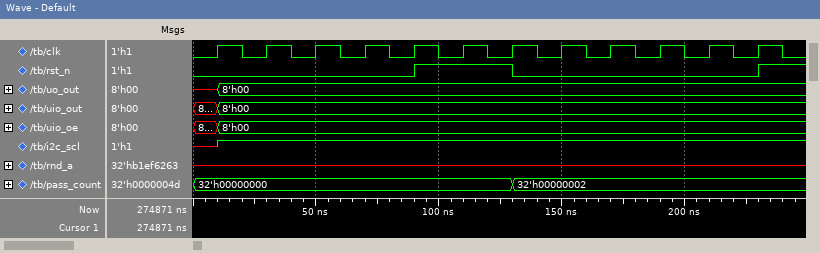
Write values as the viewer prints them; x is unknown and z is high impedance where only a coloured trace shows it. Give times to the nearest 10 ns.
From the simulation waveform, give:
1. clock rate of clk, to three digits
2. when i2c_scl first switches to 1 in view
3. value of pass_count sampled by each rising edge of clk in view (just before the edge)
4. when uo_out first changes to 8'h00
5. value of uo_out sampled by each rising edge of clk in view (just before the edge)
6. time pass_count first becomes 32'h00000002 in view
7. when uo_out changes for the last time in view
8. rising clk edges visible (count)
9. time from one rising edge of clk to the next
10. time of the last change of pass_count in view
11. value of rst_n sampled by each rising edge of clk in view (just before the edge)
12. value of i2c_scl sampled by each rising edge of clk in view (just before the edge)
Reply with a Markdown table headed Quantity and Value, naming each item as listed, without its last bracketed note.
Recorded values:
| Quantity | Value |
|---|---|
| clock rate of clk, to three digits | 50.0 MHz |
| when i2c_scl first switches to 1 in view | 10 ns |
| value of pass_count sampled by each rising edge of clk in view | 32'h00000000, 32'h00000000, 32'h00000000, 32'h00000000, 32'h00000000, 32'h00000000, 32'h00000000, 32'h00000002, 32'h00000002, 32'h00000002, 32'h00000002, 32'h00000002 |
| when uo_out first changes to 8'h00 | 10 ns |
| value of uo_out sampled by each rising edge of clk in view | x, 8'h00, 8'h00, 8'h00, 8'h00, 8'h00, 8'h00, 8'h00, 8'h00, 8'h00, 8'h00, 8'h00 |
| time pass_count first becomes 32'h00000002 in view | 130 ns |
| when uo_out changes for the last time in view | 10 ns |
| rising clk edges visible | 12 |
| time from one rising edge of clk to the next | 20 ns |
| time of the last change of pass_count in view | 130 ns |
| value of rst_n sampled by each rising edge of clk in view | 0 0 0 0 0 1 1 0 0 0 0 0 |
| value of i2c_scl sampled by each rising edge of clk in view | x 1 1 1 1 1 1 1 1 1 1 1 |
